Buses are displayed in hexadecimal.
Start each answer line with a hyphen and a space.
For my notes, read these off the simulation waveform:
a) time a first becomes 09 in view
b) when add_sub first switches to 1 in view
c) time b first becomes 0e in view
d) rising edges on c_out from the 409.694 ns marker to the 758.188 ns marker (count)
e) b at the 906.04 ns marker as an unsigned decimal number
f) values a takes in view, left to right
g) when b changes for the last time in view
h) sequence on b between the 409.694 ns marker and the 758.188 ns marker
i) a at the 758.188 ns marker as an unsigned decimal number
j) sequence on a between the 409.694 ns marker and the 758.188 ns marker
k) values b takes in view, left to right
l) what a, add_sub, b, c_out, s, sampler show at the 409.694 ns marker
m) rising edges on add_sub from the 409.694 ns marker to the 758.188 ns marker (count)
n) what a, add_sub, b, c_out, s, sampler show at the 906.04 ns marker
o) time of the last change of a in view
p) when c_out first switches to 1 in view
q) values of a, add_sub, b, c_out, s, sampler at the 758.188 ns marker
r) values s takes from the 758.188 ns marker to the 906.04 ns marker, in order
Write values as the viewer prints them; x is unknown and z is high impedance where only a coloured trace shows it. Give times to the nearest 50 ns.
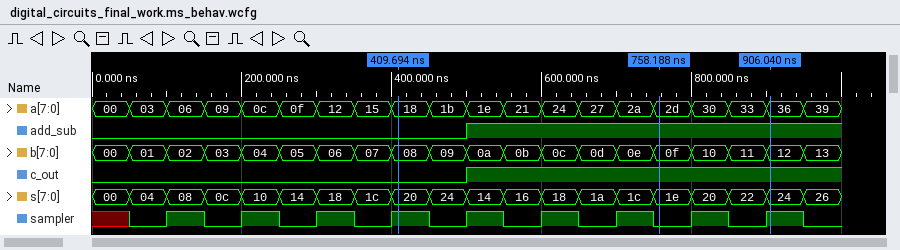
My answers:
- 150 ns
- 500 ns
- 700 ns
- 1
- 18
- 00, 03, 06, 09, 0c, 0f, 12, 15, 18, 1b, 1e, 21, 24, 27, 2a, 2d, 30, 33, 36, 39
- 950 ns
- 08, 09, 0a, 0b, 0c, 0d, 0e, 0f
- 45
- 18, 1b, 1e, 21, 24, 27, 2a, 2d
- 00, 01, 02, 03, 04, 05, 06, 07, 08, 09, 0a, 0b, 0c, 0d, 0e, 0f, 10, 11, 12, 13
- a=18, add_sub=0, b=08, c_out=0, s=20, sampler=1
- 1
- a=36, add_sub=1, b=12, c_out=1, s=24, sampler=1
- 950 ns
- 500 ns
- a=2d, add_sub=1, b=0f, c_out=1, s=1e, sampler=0
- 1e, 20, 22, 24
